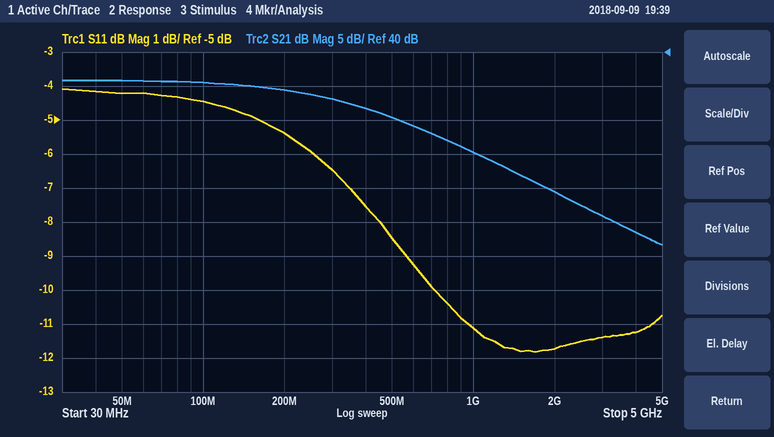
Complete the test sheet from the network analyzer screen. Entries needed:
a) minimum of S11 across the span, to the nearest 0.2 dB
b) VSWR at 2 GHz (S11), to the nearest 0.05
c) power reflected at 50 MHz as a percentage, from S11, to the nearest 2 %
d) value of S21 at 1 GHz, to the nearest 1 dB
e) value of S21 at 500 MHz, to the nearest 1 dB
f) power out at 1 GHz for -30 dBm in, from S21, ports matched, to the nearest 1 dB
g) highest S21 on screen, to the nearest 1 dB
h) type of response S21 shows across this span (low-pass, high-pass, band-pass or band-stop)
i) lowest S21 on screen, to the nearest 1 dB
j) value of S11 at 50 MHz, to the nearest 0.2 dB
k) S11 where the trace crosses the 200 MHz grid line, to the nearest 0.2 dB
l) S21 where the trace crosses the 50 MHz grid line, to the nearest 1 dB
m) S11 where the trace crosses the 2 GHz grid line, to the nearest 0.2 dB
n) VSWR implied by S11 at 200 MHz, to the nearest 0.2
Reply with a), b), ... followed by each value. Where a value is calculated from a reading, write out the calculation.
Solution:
a) -11.8 dB
b) |Γ| = 10^(-11.8/20) = 0.2570; VSWR = (1 + 0.2570)/(1 − 0.2570) ≈ 1.69, so 1.70 to the nearest 0.05
c) 10^(-4.2/10) ≈ 38 %
d) 25 dB
e) 30 dB
f) -30 dBm + (25 dB) = -5 dBm
g) 36 dB
h) low-pass
i) 12 dB
j) -4.2 dB
k) -5.4 dB
l) 36 dB
m) -11.8 dB
n) |Γ| = 10^(-5.4/20) = 0.5370; VSWR = (1 + 0.5370)/(1 − 0.5370) ≈ 3.32, so 3.4 to the nearest 0.2
